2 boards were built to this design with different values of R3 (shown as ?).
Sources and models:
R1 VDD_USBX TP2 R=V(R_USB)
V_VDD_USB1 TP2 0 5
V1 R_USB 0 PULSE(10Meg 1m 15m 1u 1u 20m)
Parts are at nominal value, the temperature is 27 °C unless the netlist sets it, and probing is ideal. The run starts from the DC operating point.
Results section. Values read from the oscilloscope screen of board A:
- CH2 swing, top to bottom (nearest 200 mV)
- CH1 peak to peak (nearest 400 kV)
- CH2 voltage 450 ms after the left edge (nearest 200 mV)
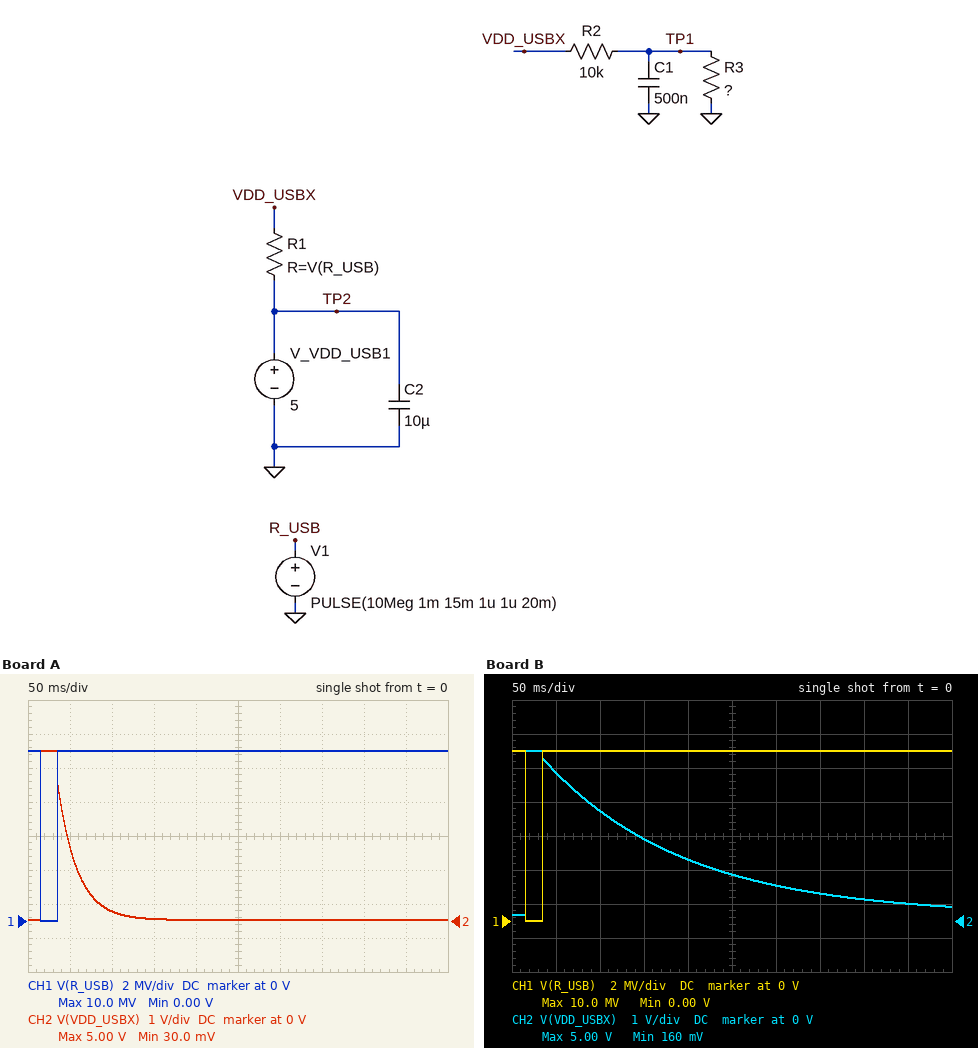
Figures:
5.0 V
10.0 MV
0 V
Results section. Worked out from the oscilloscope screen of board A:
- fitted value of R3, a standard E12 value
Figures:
47 kΩ
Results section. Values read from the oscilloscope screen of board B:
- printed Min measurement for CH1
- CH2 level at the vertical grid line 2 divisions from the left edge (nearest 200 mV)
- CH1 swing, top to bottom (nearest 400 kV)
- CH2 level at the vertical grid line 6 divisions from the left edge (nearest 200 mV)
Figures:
0.00 V
3.2 V
10.0 MV
1.0 V
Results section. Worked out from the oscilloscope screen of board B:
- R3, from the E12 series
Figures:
330 kΩ
